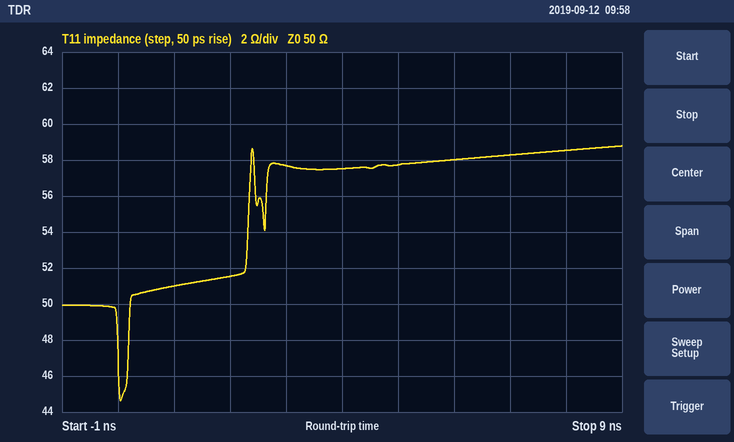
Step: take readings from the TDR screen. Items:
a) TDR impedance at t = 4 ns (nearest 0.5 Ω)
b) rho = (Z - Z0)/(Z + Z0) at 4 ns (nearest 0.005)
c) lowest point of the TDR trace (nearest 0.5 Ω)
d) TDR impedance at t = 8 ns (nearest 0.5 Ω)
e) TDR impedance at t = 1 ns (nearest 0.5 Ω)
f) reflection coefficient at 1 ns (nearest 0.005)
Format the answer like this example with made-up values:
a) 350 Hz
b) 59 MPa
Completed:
a) 57.5 Ω
b) +0.070
c) 44.5 Ω
d) 58.5 Ω
e) 51.0 Ω
f) +0.010
